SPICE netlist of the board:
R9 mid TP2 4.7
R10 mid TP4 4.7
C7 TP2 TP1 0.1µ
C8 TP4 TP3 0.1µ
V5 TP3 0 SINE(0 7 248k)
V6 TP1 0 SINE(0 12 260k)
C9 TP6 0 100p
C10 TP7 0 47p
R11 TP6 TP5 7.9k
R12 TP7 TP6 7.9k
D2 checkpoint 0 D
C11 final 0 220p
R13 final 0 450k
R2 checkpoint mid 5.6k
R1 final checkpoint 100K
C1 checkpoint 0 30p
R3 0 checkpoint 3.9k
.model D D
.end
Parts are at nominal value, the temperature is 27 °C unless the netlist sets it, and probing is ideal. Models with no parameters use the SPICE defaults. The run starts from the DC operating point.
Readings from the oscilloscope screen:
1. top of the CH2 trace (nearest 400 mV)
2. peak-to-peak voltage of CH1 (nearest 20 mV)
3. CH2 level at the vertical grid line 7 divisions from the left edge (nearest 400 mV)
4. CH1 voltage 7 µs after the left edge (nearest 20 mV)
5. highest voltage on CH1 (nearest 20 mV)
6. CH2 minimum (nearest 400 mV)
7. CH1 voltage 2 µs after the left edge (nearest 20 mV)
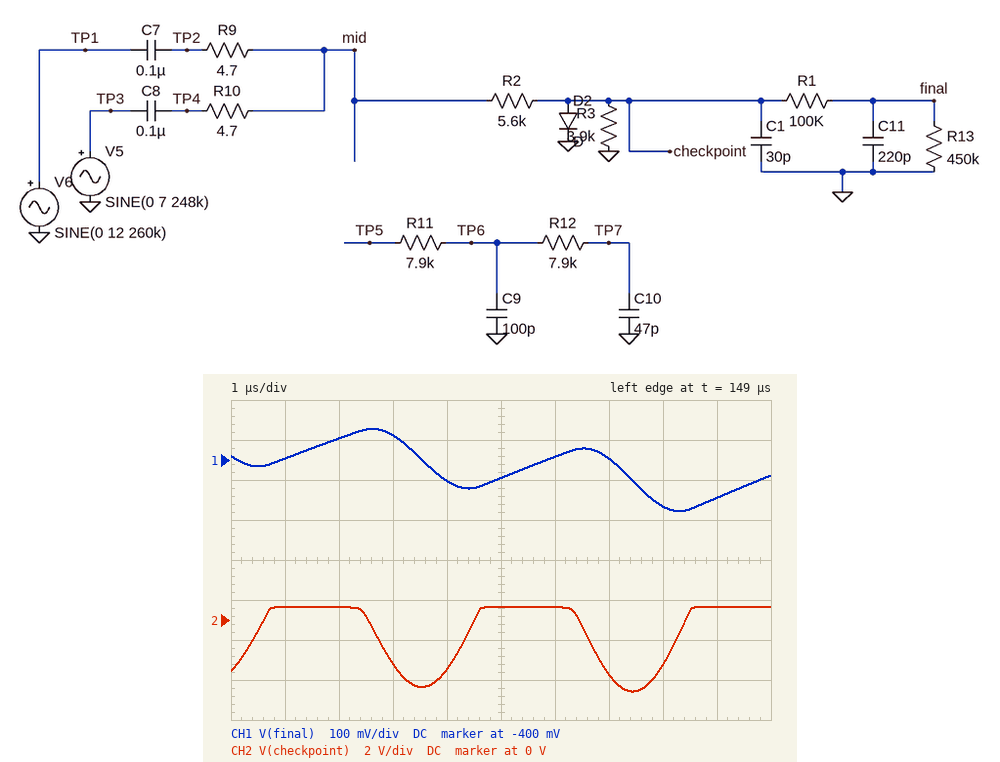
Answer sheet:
800 mV
200 mV
-2.8 V
-400 mV
-320 mV
-3.6 V
-340 mV
